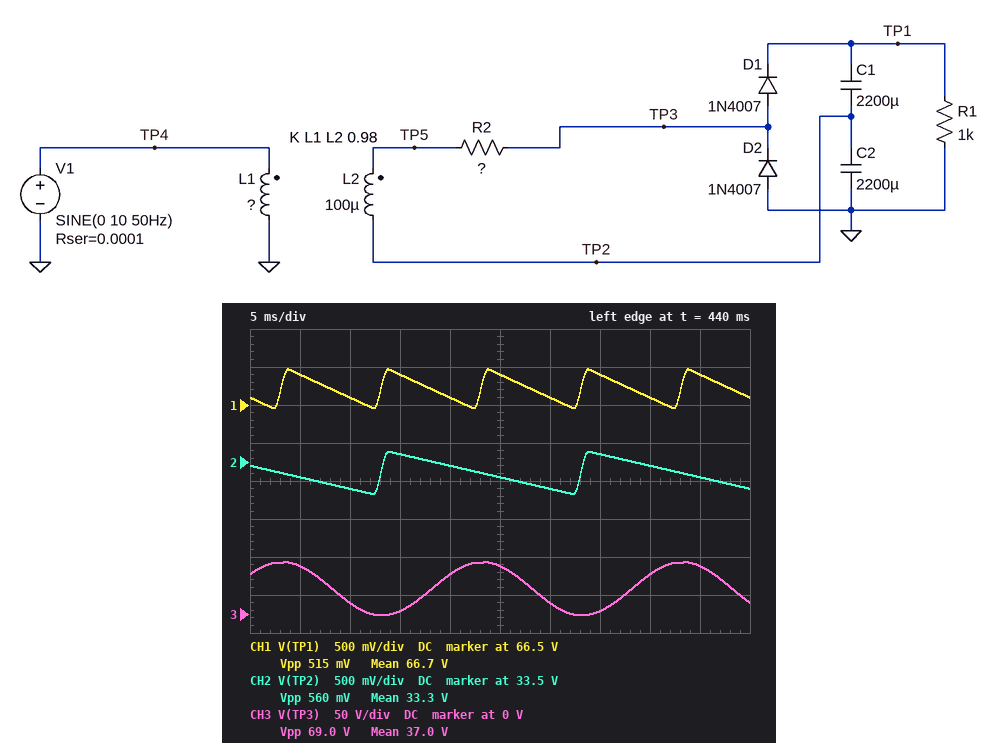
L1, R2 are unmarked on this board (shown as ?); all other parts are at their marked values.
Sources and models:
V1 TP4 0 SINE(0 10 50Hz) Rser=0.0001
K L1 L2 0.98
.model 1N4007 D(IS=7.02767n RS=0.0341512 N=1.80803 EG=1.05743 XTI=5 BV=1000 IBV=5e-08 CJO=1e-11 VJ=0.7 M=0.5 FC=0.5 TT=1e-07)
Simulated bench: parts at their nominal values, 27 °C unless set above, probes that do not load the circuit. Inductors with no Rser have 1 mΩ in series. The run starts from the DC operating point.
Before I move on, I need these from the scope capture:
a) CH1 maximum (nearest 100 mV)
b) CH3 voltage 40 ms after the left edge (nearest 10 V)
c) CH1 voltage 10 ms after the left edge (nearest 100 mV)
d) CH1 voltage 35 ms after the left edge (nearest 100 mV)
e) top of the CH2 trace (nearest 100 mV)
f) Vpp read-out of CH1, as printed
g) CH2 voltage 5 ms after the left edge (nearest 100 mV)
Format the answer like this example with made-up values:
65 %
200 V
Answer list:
67.0 V
50 V
66.6 V
66.9 V
33.6 V
515 mV
33.3 V
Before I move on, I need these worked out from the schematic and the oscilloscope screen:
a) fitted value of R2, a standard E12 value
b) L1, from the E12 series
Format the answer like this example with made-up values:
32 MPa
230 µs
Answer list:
0.56 Ω
5.6 µH
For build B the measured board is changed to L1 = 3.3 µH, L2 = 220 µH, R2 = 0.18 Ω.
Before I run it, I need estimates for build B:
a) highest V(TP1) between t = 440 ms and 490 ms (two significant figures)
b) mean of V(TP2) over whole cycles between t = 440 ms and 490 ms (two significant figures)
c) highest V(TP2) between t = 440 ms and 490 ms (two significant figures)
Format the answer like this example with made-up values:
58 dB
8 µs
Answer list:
110 V
53 V
54 V
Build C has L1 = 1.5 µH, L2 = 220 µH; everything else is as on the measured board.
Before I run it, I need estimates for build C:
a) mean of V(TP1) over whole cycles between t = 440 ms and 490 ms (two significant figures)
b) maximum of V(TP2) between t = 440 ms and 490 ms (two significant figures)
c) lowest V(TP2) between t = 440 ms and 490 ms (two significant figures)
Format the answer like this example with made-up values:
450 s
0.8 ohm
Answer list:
89 V
45 V
44 V
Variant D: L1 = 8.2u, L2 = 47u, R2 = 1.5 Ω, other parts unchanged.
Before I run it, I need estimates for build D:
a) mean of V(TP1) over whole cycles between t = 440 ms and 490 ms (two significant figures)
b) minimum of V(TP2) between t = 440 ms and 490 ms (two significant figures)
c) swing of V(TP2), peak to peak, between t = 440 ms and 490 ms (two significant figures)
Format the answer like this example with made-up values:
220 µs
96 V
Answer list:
40 V
20 V
320 mV
